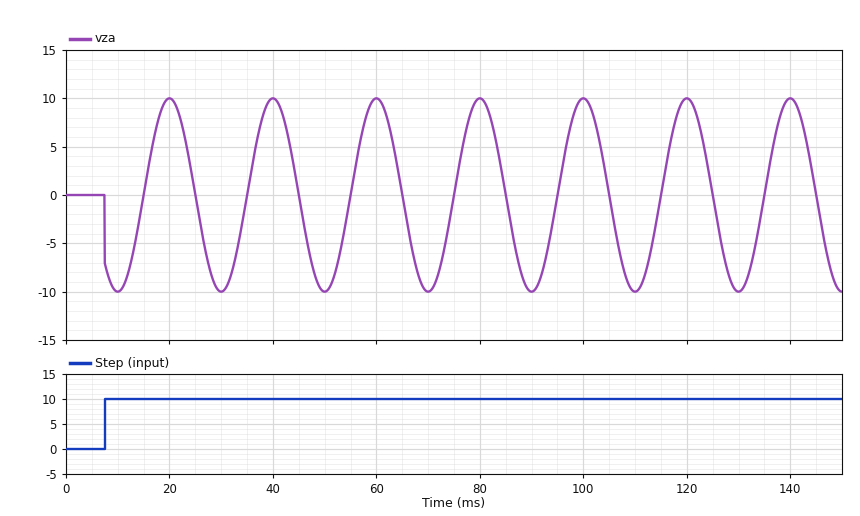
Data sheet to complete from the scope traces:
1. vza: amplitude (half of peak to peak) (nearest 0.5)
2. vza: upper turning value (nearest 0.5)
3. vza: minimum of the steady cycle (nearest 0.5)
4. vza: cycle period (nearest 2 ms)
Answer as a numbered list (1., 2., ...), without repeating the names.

1. 10.0
2. 10.0
3. -10.0
4. 20 ms
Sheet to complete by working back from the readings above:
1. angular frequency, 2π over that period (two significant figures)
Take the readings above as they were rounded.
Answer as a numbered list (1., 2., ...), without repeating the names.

1. 0.31 rad/ms
